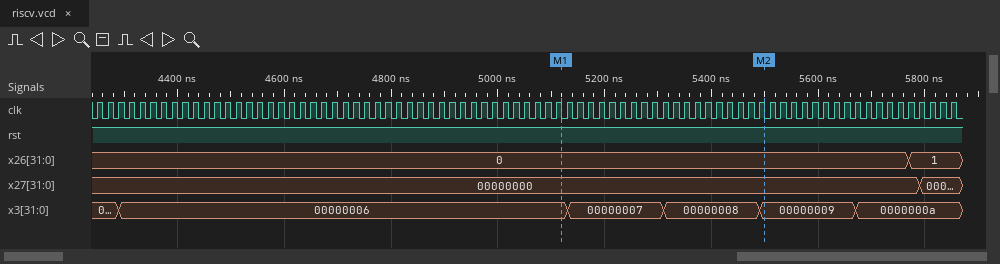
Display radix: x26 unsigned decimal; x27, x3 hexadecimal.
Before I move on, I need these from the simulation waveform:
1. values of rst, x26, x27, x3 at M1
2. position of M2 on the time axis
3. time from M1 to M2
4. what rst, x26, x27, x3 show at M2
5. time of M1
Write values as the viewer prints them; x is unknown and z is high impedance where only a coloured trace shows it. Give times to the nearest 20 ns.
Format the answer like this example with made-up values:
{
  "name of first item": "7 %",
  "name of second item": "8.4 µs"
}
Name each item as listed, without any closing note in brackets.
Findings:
{
  "values of rst, x26, x27, x3 at M1": "rst=1, x26=0, x27=00000000, x3=00000006",
  "position of M2 on the time axis": "5500 ns",
  "time from M1 to M2": "380 ns",
  "what rst, x26, x27, x3 show at M2": "rst=1, x26=0, x27=00000000, x3=00000009",
  "time of M1": "5120 ns"
}
